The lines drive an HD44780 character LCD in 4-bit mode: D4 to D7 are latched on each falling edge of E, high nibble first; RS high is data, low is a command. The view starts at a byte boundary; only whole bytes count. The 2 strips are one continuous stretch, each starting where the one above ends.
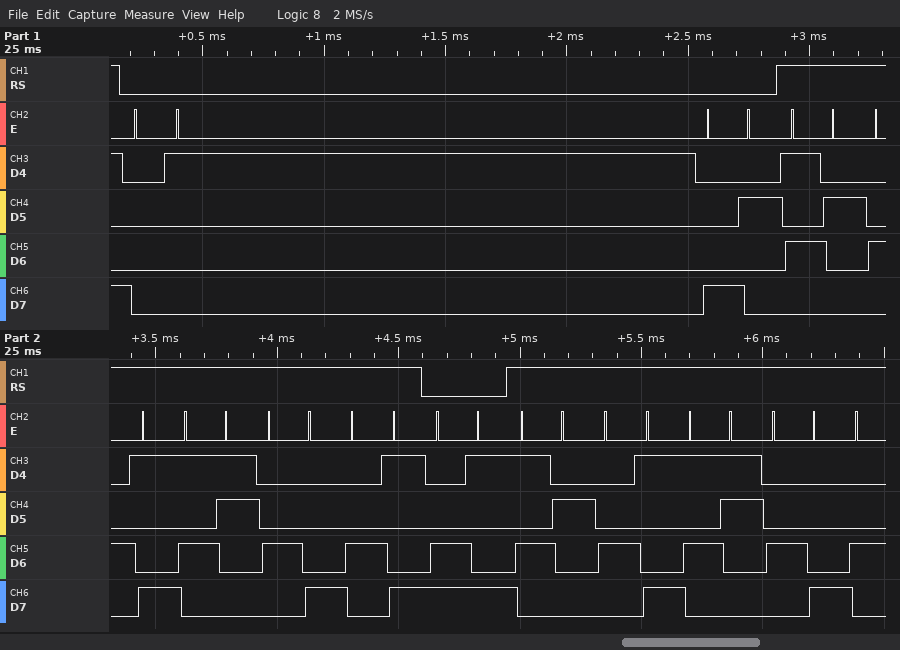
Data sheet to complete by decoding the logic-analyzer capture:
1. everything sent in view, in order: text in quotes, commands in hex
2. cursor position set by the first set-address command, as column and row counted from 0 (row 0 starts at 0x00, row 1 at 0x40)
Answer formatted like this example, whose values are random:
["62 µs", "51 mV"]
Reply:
["0x01 0x82 \"RISHI\" 0xC9 \"RISH\"", "column 2, row 0"]
